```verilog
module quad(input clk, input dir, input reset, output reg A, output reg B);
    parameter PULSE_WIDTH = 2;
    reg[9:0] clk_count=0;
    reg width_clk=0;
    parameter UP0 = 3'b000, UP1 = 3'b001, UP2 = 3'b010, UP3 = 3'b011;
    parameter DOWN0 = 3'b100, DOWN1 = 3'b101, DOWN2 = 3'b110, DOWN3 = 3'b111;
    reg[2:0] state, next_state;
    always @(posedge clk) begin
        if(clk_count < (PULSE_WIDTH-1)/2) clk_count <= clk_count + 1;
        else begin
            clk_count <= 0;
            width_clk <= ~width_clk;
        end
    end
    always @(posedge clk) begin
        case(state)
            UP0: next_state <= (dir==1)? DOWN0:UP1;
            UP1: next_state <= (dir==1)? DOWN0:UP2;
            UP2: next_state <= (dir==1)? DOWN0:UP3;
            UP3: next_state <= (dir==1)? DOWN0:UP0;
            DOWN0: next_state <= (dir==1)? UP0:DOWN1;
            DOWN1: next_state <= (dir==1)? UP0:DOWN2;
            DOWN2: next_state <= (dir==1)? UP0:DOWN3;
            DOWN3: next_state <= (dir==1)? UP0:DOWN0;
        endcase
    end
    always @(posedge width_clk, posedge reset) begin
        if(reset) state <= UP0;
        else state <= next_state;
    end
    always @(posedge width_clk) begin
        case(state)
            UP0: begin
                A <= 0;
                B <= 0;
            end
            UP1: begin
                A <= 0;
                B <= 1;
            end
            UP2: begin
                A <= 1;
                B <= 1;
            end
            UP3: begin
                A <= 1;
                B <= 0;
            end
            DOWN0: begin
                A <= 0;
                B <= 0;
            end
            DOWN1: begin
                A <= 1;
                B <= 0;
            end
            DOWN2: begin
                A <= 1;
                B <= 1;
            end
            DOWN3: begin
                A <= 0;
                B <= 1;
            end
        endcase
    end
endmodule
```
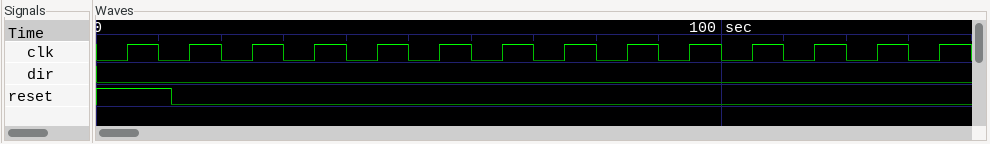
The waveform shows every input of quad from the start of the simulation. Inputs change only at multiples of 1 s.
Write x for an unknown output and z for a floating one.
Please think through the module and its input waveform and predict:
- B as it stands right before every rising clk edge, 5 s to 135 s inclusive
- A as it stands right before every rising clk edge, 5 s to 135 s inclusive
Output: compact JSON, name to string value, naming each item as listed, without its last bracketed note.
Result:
{"B as it stands right before every rising clk edge, 5 s to 135 s inclusive": "x 0 0 0 0 1 1 1 1 0 0 0 0 1", "A as it stands right before every rising clk edge, 5 s to 135 s inclusive": "x 0 0 0 0 0 0 1 1 1 1 0 0 0"}
